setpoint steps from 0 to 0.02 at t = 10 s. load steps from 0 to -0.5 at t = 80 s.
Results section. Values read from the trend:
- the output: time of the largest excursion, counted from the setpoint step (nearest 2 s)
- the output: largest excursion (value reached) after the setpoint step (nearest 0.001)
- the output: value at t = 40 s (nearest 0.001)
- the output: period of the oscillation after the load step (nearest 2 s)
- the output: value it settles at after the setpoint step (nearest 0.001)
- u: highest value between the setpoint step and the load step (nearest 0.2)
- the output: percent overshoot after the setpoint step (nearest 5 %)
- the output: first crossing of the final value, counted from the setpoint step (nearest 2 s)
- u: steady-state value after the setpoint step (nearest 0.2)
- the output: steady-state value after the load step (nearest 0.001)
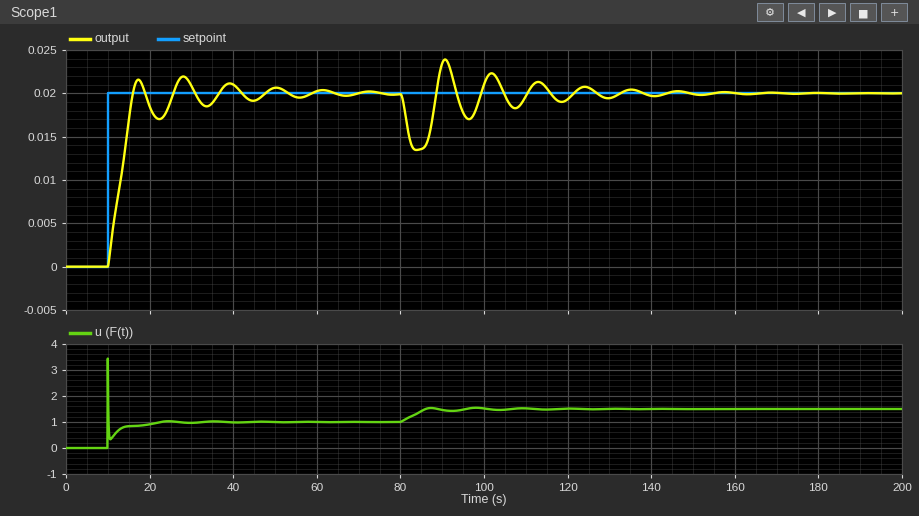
18 s
0.022
0.021
12 s
0.020
3.4
10 %
6 s
1.0
0.020
